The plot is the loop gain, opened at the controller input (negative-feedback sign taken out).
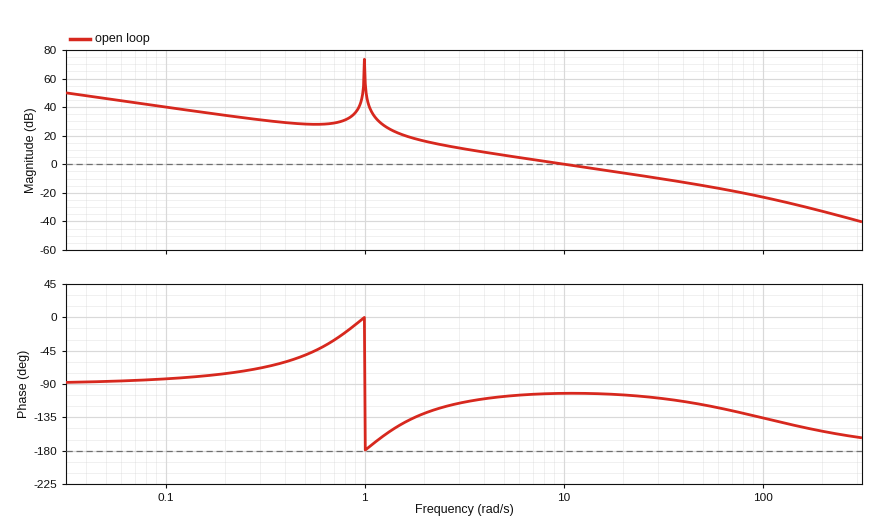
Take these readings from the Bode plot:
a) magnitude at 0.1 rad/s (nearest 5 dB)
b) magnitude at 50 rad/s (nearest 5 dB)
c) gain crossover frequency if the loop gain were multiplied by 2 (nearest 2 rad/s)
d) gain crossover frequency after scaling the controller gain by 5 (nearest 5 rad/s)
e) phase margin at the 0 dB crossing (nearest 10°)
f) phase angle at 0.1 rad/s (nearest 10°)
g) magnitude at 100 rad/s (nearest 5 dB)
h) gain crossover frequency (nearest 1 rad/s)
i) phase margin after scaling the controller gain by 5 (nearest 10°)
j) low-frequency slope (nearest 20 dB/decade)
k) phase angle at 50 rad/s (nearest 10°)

40 dB
-15 dB
20 rad/s
45 rad/s
80°
-80°
-25 dB
10 rad/s
60°
-20 dB/decade
-120°
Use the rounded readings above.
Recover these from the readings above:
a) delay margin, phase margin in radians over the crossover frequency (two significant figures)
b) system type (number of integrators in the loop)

0.14 s
1
